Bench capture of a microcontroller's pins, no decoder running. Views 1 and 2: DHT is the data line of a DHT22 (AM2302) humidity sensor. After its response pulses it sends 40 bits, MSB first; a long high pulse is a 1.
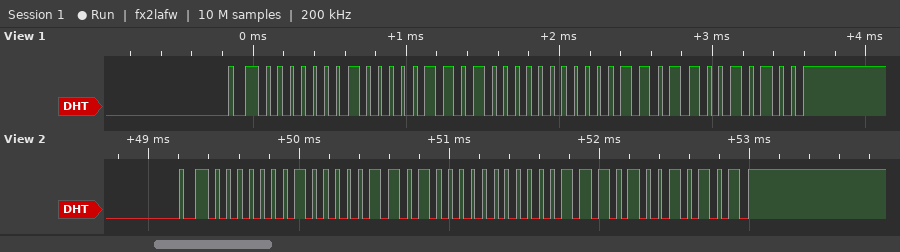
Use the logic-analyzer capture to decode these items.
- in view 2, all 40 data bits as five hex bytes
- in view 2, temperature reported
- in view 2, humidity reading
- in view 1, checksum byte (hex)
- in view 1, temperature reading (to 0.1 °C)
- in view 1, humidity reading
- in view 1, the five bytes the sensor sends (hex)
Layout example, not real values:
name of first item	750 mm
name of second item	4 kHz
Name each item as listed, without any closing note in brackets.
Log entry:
in view 2, all 40 data bits as five hex bytes	01 06 80 0E 95
in view 2, temperature reported	-1.4 °C
in view 2, humidity reading	26.2 %
in view 1, checksum byte	0x94
in view 1, temperature reading	-1.3 °C
in view 1, humidity reading	26.2 %
in view 1, the five bytes the sensor sends	01 06 80 0D 94
